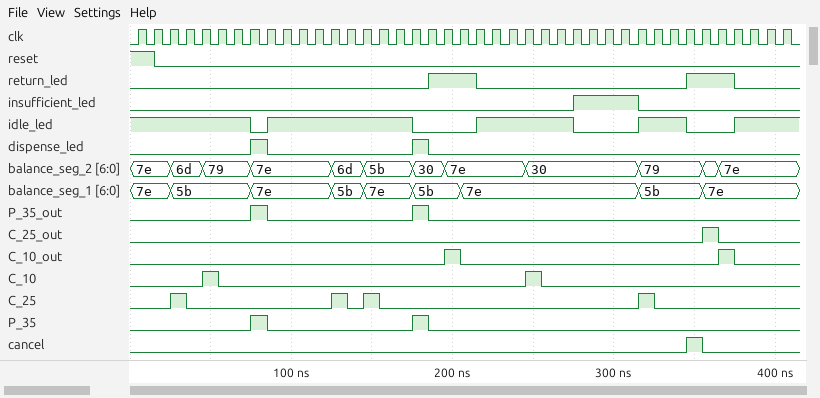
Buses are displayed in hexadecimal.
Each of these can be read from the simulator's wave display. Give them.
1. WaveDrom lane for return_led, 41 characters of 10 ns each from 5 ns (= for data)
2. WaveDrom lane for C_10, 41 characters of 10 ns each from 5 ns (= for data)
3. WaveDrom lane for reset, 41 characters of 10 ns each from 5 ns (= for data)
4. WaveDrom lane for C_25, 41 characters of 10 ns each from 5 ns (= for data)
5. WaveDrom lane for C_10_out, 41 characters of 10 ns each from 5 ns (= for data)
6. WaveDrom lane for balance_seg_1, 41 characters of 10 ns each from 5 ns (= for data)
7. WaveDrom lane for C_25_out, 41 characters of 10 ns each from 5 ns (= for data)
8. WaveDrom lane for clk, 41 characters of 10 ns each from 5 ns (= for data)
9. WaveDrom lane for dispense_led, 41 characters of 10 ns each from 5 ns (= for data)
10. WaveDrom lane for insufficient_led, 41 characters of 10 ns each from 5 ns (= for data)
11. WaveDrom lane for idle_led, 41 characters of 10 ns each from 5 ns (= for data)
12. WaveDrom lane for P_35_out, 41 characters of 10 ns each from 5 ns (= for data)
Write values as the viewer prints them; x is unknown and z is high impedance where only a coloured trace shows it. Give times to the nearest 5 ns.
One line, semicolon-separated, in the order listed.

{name: 'return_led', wave: '0.................1..0............1..0...'}; {name: 'C_10', wave: '0...10..................10...............'}; {name: 'reset', wave: '10.......................................'}; {name: 'C_25', wave: '0.10........1010...............10........'}; {name: 'C_10_out', wave: '0..................10...............10...'}; {name: 'balance_seg_1', wave: '=.=....=....=.=..=..=..........=...=.....', data: '7e 5b 7e 5b 7e 5b 7e 5b 7e'}; {name: 'C_25_out', wave: '0..................................10....'}; {name: 'clk', wave: 'p........................................'}; {name: 'dispense_led', wave: '0......10........10......................'}; {name: 'insufficient_led', wave: '0..........................1...0.........'}; {name: 'idle_led', wave: '1......01........0...1.....0...1..0..1...'}; {name: 'P_35_out', wave: '0......10........10......................'}
